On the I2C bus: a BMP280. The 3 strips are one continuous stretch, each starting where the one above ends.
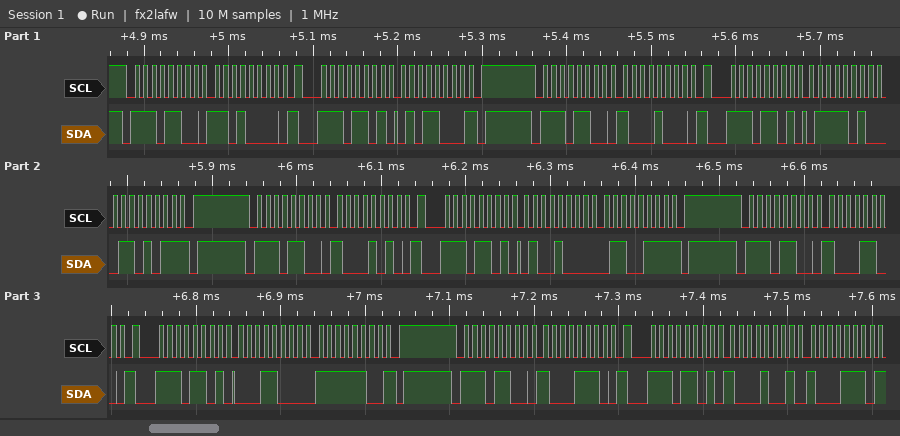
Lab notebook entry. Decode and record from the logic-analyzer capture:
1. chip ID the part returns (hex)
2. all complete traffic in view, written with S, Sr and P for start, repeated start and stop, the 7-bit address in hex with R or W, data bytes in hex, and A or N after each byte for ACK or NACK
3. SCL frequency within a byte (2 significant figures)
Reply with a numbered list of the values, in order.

1. 0x58
2. S 76W A D0 A Sr 76R A 58 N P S 76W A 88 A Sr 76R A 7A A 6B N P S 76W A 8A A Sr 76R A 48 A 67 N P S 76W A 8C A Sr 76R A 18 A FC N P S 76W A 8E A Sr 76R A 89 A 8E N
3. 100 kHz
